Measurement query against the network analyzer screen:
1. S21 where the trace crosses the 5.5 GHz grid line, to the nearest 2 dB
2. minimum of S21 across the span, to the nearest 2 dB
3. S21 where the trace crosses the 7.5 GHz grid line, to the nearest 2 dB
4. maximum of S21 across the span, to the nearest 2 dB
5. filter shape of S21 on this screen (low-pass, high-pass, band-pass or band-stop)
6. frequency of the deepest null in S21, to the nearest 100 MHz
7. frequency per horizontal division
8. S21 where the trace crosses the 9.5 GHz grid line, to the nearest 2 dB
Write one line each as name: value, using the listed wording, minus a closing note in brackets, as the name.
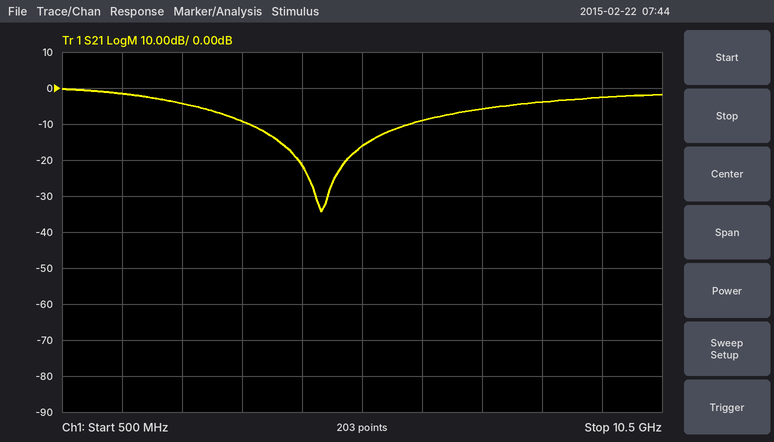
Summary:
S21 where the trace crosses the 5.5 GHz grid line, to the nearest 2 dB: -16 dB
minimum of S21 across the span, to the nearest 2 dB: -34 dB
S21 where the trace crosses the 7.5 GHz grid line, to the nearest 2 dB: -6 dB
maximum of S21 across the span, to the nearest 2 dB: 0 dB
filter shape of S21 on this screen: band-stop
frequency of the deepest null in S21, to the nearest 100 MHz: 4.8 GHz
frequency per horizontal division: 1 GHz
S21 where the trace crosses the 9.5 GHz grid line, to the nearest 2 dB: -2 dB
